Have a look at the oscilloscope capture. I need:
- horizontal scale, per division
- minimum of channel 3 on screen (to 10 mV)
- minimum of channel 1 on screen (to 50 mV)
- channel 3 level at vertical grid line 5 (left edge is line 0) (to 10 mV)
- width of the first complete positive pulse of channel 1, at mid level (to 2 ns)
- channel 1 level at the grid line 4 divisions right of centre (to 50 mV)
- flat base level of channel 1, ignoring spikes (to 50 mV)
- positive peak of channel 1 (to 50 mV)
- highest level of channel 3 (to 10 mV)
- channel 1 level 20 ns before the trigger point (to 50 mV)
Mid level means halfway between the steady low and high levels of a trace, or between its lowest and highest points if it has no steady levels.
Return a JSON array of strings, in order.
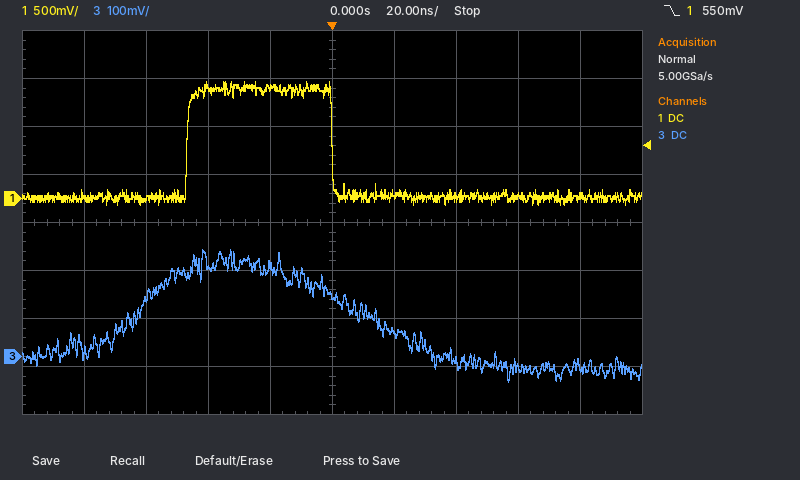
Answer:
["20 ns", "-50 mV", "-50 mV", "130 mV", "46 ns", "0 mV", "0 mV", "1.20 V", "220 mV", "1.15 V"]
